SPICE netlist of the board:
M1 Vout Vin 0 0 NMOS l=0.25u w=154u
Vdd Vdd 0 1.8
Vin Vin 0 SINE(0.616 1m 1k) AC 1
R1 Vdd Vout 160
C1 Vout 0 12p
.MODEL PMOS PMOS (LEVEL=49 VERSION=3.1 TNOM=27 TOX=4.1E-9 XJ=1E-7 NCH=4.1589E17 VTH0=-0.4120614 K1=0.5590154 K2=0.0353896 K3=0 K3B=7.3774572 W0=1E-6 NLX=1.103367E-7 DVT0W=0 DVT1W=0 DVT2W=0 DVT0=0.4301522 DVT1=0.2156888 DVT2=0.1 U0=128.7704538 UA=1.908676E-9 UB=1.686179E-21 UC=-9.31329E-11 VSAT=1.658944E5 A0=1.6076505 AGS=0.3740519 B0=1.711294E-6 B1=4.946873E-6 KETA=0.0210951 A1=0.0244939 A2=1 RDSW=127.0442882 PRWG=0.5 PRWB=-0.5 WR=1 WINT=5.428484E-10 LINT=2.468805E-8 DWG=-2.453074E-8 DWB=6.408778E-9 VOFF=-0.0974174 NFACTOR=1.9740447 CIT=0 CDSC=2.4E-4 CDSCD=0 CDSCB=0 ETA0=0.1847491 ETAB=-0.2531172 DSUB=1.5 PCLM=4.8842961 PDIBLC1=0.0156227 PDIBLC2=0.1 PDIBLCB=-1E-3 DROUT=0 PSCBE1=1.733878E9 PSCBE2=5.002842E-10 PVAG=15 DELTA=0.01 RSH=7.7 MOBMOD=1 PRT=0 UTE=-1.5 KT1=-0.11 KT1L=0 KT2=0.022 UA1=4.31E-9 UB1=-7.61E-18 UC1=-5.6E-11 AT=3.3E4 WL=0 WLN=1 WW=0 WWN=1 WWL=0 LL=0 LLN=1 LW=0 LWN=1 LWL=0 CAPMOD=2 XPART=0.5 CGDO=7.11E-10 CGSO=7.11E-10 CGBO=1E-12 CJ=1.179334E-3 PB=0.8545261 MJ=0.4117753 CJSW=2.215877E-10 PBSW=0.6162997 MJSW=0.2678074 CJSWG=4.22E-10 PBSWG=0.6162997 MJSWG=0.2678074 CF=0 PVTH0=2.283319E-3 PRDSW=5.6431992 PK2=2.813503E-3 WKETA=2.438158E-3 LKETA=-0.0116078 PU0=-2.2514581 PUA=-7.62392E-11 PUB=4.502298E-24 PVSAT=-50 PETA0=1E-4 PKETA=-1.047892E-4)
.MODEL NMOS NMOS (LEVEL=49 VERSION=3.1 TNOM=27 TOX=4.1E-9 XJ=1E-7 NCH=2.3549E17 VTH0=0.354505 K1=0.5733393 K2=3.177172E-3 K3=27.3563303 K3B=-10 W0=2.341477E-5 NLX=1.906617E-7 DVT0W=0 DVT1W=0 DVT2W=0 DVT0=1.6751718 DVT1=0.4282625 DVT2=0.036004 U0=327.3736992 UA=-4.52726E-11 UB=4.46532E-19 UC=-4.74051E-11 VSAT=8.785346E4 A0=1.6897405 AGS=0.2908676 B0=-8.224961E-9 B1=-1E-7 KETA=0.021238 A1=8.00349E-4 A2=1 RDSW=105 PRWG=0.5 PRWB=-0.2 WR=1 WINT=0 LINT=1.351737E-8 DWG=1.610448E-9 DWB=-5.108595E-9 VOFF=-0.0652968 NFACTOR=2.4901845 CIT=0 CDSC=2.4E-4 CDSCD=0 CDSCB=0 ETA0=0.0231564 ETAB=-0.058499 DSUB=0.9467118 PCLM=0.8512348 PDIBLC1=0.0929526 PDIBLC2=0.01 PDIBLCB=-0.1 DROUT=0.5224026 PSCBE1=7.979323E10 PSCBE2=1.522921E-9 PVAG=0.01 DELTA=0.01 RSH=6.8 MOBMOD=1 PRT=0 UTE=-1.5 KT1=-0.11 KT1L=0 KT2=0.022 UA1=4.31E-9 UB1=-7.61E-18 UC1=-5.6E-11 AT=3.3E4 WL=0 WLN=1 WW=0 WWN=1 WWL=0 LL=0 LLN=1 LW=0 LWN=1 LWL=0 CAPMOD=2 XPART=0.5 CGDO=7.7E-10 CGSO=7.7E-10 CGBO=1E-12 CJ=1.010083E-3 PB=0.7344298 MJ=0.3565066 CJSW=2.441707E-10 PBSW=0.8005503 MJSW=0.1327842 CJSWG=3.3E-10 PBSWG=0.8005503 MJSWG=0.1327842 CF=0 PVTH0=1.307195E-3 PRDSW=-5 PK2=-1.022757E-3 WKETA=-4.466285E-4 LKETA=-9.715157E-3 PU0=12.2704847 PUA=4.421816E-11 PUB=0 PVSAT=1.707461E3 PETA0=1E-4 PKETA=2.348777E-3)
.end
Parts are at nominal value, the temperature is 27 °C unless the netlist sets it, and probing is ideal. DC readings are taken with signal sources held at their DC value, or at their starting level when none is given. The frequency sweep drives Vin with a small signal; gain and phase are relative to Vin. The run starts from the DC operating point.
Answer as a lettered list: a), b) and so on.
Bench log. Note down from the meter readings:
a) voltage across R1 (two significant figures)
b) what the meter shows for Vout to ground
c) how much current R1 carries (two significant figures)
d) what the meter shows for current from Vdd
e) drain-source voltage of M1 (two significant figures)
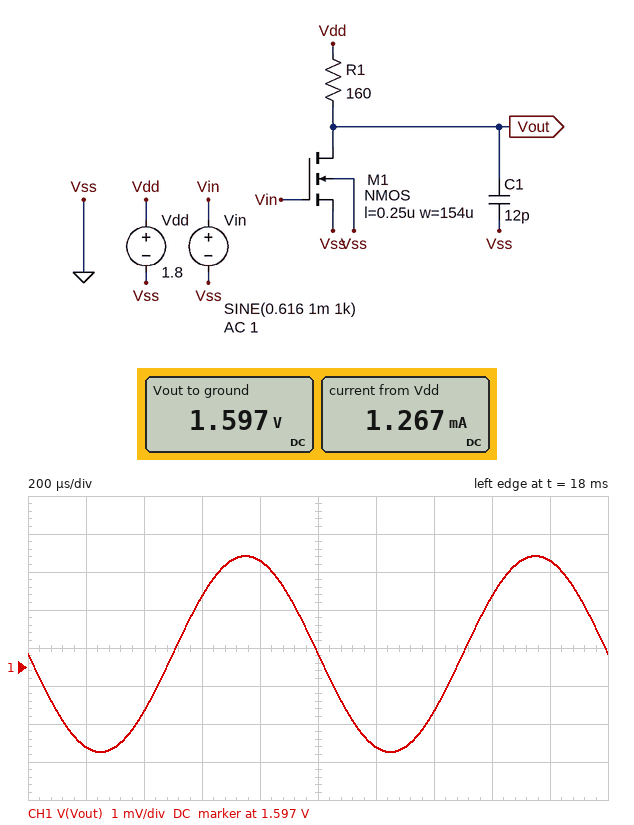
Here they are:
a) 200 mV
b) 1.597 V
c) 1.3 mA
d) 1.267 mA
e) 1.6 V
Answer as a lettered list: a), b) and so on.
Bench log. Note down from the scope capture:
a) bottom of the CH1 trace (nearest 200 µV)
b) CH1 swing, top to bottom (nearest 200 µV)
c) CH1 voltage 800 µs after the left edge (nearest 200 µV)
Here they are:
a) 1.5948 V
b) 5.2 mV
c) 1.5998 V
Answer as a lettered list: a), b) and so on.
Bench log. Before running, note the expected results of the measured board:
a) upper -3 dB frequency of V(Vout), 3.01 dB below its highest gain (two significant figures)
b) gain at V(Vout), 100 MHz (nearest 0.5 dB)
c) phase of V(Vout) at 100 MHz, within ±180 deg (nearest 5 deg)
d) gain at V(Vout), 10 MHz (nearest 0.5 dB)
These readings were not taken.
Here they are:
a) 84 MHz
b) 4.5 dB
c) 130 deg
d) 8.0 dB
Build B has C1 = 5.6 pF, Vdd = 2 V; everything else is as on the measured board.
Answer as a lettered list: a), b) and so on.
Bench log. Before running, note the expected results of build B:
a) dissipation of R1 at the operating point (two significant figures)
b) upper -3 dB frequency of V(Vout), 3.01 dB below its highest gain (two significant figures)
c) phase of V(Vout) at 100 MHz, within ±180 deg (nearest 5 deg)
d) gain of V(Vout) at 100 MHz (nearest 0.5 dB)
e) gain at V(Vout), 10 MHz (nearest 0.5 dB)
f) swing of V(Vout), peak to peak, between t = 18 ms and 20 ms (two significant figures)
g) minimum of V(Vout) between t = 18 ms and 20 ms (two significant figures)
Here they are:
a) 270 µW
b) 180 MHz
c) 150 deg
d) 7.0 dB
e) 8.5 dB
f) 5.3 mV
g) 1.8 V
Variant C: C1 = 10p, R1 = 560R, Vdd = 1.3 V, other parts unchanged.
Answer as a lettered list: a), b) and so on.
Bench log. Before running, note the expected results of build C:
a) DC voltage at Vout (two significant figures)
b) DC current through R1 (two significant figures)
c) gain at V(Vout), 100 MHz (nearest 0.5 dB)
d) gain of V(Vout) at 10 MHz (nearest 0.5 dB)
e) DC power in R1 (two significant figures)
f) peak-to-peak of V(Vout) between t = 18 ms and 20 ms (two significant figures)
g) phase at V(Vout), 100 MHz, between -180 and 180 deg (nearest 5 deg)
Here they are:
a) 690 mV
b) 1.1 mA
c) 7.0 dB
d) 17.0 dB
e) 660 µW
f) 15 mV
g) 105 deg
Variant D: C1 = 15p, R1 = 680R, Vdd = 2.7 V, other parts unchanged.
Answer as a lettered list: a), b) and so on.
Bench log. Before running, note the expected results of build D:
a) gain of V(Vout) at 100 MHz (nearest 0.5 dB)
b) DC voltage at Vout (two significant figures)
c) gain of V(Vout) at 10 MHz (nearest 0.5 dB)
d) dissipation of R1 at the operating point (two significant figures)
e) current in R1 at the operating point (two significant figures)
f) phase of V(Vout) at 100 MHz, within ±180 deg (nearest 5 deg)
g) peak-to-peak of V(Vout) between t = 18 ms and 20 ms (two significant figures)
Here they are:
a) 5.0 dB
b) 1.8 V
c) 19.0 dB
d) 1.2 mW
e) 1.3 mA
f) 100 deg
g) 20 mV
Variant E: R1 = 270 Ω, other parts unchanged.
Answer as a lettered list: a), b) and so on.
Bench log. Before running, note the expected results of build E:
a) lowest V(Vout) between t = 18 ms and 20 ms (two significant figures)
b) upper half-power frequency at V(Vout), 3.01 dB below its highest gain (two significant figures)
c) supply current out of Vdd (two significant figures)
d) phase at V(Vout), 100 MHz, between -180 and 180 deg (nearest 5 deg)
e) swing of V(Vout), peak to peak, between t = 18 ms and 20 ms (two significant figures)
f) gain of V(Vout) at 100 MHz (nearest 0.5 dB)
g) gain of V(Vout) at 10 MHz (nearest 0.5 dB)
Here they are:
a) 1.5 V
b) 51 MHz
c) 1.2 mA
d) 115 deg
e) 8.4 mV
f) 5.5 dB
g) 12.5 dB
